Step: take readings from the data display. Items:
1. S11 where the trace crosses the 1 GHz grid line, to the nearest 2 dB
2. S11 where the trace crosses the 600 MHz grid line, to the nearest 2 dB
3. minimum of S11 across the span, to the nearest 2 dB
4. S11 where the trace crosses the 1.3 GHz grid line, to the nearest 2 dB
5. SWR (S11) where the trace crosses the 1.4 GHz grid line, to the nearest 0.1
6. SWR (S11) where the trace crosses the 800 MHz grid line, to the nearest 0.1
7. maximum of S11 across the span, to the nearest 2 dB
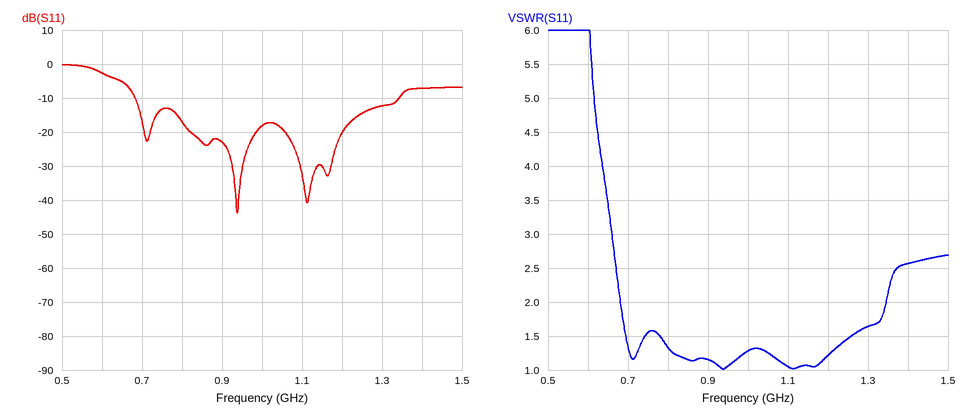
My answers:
-18 dB
-2 dB
-44 dB
-12 dB
2.6
1.3
0 dB
